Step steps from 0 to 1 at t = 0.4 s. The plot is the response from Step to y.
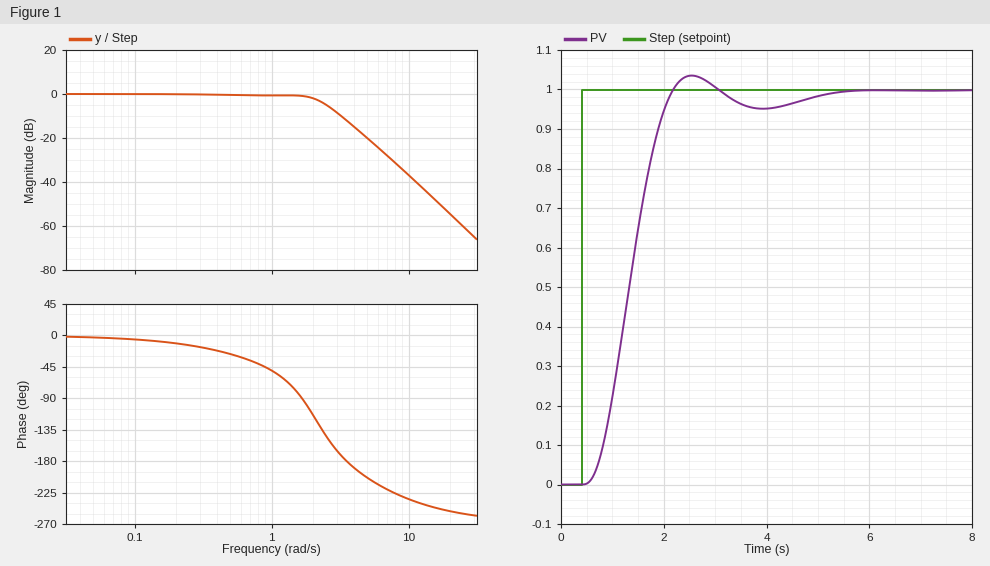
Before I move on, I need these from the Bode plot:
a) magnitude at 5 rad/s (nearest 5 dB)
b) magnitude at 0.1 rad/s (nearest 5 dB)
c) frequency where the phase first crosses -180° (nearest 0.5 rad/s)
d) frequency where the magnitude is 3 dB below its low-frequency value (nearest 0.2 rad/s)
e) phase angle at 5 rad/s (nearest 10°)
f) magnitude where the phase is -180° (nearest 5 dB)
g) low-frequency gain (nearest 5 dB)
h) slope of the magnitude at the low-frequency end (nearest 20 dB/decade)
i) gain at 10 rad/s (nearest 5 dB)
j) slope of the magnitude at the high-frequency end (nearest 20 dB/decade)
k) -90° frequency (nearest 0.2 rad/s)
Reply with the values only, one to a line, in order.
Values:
-20 dB
0 dB
3.5 rad/s
2.2 rad/s
-200°
-10 dB
0 dB
0 dB/decade
-35 dB
-60 dB/decade
1.6 rad/s
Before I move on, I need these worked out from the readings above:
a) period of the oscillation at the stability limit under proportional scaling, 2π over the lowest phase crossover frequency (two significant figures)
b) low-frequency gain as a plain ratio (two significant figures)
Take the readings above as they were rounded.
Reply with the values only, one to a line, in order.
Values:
1.8 s
1.0
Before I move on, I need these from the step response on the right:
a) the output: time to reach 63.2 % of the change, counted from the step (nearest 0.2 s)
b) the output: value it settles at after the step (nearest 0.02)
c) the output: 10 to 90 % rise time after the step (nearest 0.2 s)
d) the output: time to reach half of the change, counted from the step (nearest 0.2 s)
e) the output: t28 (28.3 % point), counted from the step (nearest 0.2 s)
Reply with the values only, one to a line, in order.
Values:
1.0 s
1.00
1.0 s
1.0 s
0.6 s
